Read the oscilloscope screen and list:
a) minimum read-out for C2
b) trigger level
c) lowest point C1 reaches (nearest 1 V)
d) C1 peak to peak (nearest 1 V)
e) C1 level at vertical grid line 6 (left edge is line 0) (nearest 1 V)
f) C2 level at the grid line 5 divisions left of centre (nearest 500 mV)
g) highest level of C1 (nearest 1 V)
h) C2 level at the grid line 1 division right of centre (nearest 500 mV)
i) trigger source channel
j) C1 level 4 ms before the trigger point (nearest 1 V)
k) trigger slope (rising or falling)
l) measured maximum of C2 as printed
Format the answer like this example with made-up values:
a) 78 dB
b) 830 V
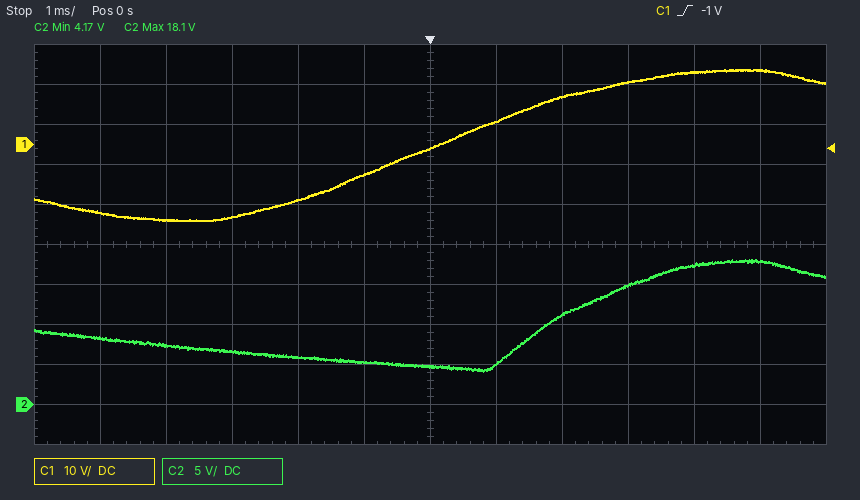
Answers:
a) 4.17 V
b) -1 V
c) -19 V
d) 38 V
e) -1 V
f) 8.5 V
g) 19 V
h) 5.0 V
i) C1
j) -19 V
k) rising
l) 18.1 V
